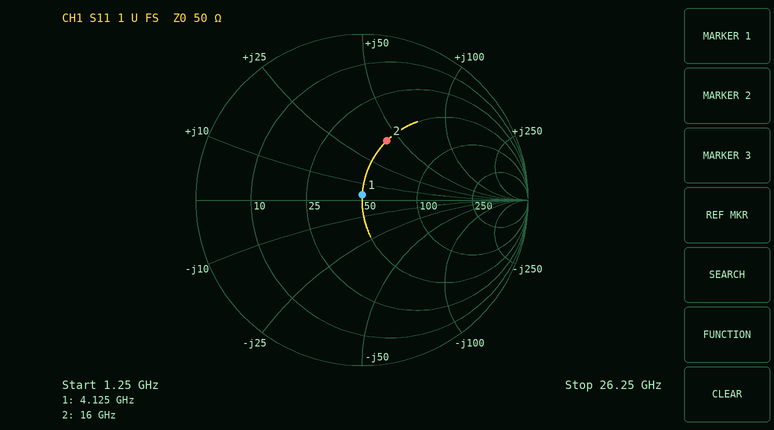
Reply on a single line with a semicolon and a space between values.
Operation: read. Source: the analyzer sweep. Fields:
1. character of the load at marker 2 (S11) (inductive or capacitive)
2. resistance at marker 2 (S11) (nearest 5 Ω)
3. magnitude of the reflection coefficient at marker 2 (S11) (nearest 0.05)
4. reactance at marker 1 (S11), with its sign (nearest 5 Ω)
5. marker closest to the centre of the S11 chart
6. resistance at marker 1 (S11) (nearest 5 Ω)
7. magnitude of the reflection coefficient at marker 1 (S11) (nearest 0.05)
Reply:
inductive; 50 Ω; 0.40; +5 Ω; marker 1; 50 Ω; 0.05
